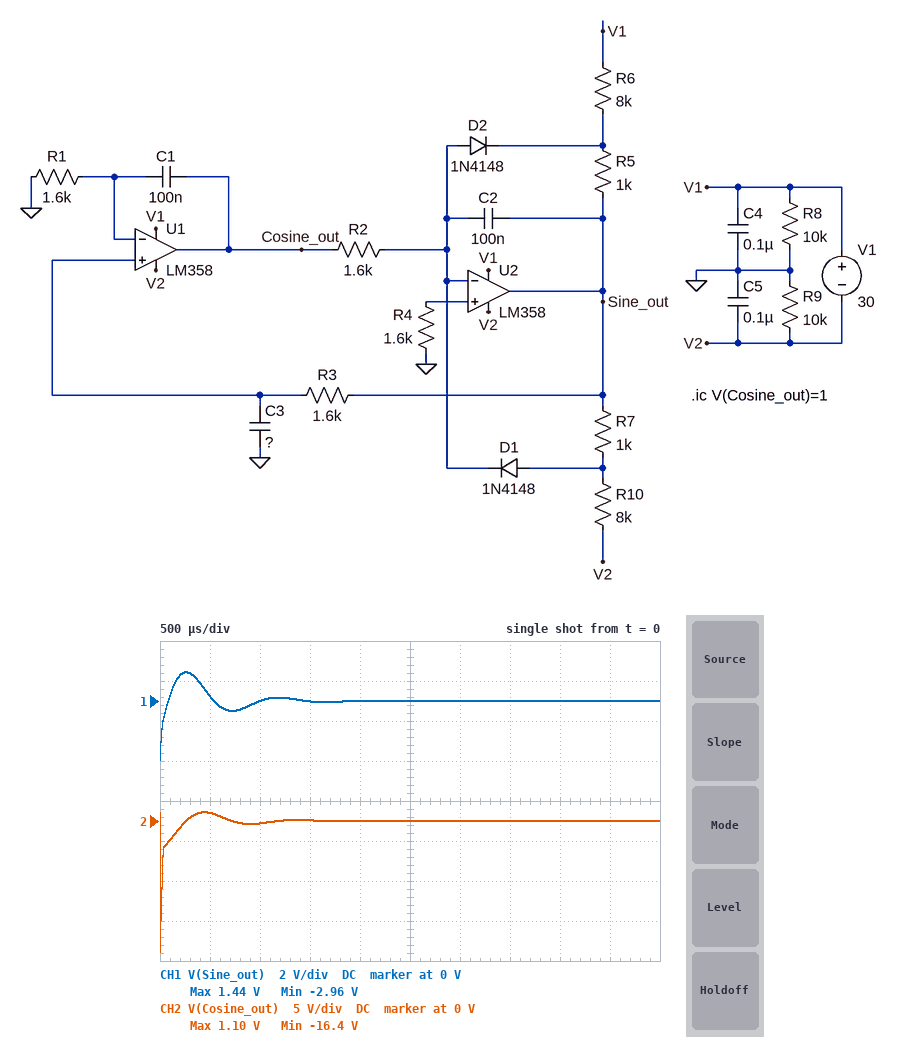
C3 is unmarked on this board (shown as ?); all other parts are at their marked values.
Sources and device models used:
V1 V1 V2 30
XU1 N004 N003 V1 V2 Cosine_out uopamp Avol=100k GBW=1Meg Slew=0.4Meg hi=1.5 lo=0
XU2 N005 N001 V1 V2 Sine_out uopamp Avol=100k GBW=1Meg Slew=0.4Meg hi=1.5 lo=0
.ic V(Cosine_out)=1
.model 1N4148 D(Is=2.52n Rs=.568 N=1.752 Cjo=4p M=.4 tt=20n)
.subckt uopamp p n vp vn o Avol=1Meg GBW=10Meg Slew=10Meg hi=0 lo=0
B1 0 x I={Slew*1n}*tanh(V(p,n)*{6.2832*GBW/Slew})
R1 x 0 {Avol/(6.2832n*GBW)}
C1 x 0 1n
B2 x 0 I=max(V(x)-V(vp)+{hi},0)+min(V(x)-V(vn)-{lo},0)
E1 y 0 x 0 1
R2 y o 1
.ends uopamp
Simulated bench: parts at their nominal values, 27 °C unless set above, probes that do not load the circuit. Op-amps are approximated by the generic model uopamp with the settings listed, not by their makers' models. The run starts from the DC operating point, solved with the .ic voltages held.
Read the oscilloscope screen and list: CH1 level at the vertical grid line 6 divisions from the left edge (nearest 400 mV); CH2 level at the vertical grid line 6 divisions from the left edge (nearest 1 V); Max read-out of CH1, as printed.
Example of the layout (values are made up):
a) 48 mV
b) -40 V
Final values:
a) 0 V
b) 0 V
c) 1.44 V
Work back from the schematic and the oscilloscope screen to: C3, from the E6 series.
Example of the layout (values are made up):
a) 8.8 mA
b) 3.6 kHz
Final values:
a) 33 nF
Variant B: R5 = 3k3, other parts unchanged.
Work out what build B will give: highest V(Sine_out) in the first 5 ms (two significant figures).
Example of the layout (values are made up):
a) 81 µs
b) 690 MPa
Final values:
a) 3.6 V
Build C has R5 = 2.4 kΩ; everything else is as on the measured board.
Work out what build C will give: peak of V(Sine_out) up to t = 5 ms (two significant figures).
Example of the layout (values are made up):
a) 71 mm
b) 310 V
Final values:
a) 2.9 V
